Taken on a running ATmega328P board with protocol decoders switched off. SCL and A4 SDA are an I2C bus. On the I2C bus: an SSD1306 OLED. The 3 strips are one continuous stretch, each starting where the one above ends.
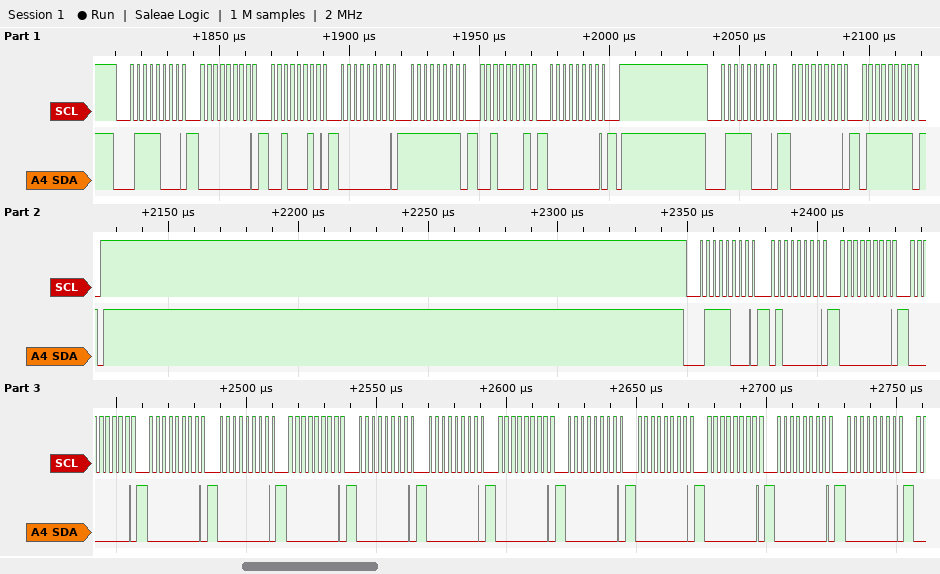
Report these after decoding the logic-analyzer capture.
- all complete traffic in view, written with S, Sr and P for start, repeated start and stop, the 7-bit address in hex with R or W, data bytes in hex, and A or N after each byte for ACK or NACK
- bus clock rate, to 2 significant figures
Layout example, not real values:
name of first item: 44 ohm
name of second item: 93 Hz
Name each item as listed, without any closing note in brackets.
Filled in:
all complete traffic in view, written with S, Sr and P for start, repeated start and stop, the 7-bit address in hex with R or W, data bytes in hex, and A or N after each byte for ACK or NACK: S 3CW A 00 A 22 A 00 A FF A 21 A 00 A P S 3CW A 00 A 7F A P S 3CW A 40 A 00 A 00 A 00 A 00 A 00 A 00 A 00 A 00 A 00 A 00 A 00 A 00 A 00 A
bus clock rate, to 2 significant figures: 400 kHz
